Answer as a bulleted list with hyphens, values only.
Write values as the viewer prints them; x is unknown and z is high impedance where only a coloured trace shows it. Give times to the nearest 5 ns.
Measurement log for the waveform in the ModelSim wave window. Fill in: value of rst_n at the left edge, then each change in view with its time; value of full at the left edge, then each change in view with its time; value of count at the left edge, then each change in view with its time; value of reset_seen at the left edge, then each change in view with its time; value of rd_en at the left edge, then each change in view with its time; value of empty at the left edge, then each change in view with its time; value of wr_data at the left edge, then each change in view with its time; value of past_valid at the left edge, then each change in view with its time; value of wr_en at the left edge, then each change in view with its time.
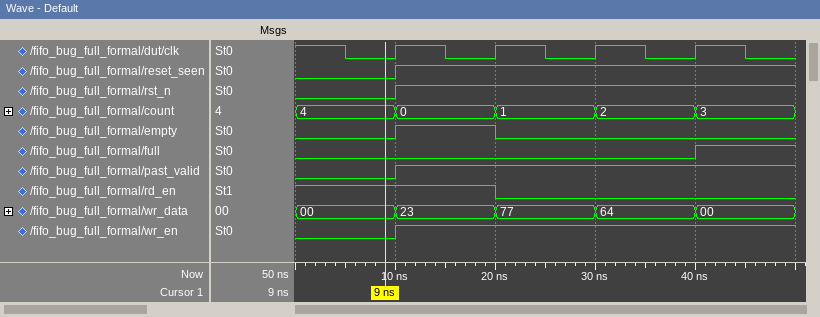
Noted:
- 0, 1 at 10 ns
- 0, 1 at 40 ns
- 4, 0 at 10 ns, 1 at 20 ns, 2 at 30 ns, 3 at 40 ns
- 0, 1 at 10 ns
- 1, 0 at 20 ns
- 0, 1 at 10 ns, 0 at 20 ns
- 00, 23 at 10 ns, 77 at 20 ns, 64 at 30 ns, 00 at 40 ns
- 0, 1 at 10 ns
- 0, 1 at 10 ns
